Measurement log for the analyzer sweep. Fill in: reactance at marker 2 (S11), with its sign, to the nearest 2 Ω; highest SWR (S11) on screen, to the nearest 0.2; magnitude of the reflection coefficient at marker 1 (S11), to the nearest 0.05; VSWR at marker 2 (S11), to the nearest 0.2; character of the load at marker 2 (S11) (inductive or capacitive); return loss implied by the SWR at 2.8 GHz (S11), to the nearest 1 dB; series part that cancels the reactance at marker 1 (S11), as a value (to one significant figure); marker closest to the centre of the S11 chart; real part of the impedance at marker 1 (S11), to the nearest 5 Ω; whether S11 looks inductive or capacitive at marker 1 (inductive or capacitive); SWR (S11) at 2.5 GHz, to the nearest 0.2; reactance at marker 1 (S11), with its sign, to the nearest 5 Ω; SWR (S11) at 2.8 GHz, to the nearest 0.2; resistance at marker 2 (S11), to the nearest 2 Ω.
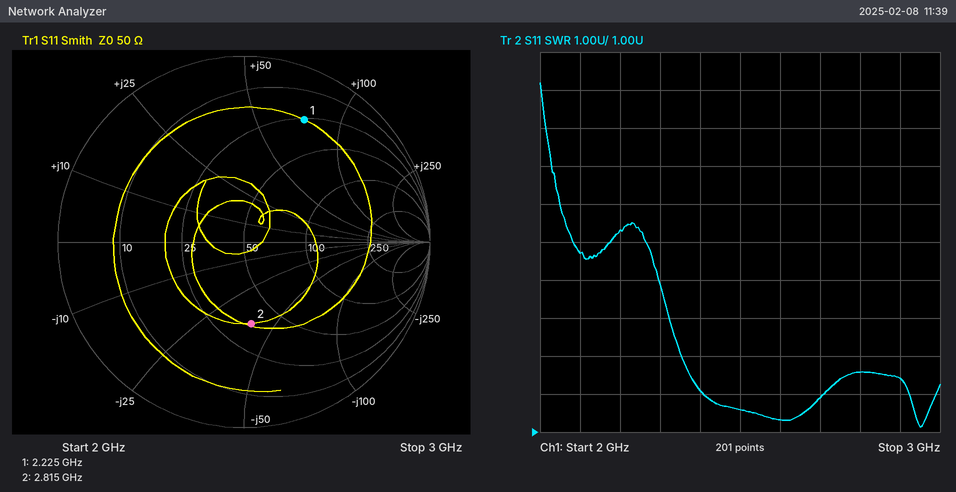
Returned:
-40 Ω
10.2
0.75
2.6
capacitive
7 dB
1.0 pF
marker 2
25 Ω
inductive
1.6
+75 Ω
2.6
36 Ω
